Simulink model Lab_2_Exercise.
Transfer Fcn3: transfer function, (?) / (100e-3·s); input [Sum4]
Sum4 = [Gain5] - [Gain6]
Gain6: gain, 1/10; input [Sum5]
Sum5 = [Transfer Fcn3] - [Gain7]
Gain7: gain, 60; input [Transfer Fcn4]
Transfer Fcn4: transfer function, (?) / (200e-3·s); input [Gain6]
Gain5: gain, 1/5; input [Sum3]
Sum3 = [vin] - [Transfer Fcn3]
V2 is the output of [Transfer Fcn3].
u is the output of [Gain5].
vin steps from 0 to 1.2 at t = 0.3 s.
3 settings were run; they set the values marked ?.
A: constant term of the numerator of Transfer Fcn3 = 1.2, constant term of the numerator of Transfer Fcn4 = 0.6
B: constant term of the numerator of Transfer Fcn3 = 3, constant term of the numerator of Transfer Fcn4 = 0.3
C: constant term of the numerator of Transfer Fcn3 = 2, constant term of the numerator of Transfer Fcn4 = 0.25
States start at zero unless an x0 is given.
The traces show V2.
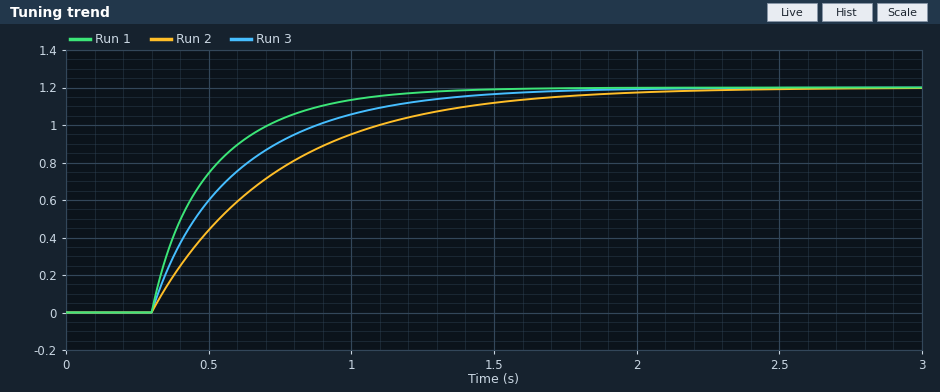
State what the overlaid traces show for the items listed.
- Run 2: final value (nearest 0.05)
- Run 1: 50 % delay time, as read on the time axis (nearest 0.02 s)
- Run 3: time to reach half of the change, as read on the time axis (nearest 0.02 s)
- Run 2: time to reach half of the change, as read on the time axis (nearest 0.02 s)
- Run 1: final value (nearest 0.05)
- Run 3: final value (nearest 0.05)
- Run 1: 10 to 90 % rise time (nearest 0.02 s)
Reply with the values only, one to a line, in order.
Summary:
1.20
0.44 s
0.50 s
0.60 s
1.20
1.20
0.52 s
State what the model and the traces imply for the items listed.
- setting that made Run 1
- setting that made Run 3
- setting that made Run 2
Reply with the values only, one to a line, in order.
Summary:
B
C
A
